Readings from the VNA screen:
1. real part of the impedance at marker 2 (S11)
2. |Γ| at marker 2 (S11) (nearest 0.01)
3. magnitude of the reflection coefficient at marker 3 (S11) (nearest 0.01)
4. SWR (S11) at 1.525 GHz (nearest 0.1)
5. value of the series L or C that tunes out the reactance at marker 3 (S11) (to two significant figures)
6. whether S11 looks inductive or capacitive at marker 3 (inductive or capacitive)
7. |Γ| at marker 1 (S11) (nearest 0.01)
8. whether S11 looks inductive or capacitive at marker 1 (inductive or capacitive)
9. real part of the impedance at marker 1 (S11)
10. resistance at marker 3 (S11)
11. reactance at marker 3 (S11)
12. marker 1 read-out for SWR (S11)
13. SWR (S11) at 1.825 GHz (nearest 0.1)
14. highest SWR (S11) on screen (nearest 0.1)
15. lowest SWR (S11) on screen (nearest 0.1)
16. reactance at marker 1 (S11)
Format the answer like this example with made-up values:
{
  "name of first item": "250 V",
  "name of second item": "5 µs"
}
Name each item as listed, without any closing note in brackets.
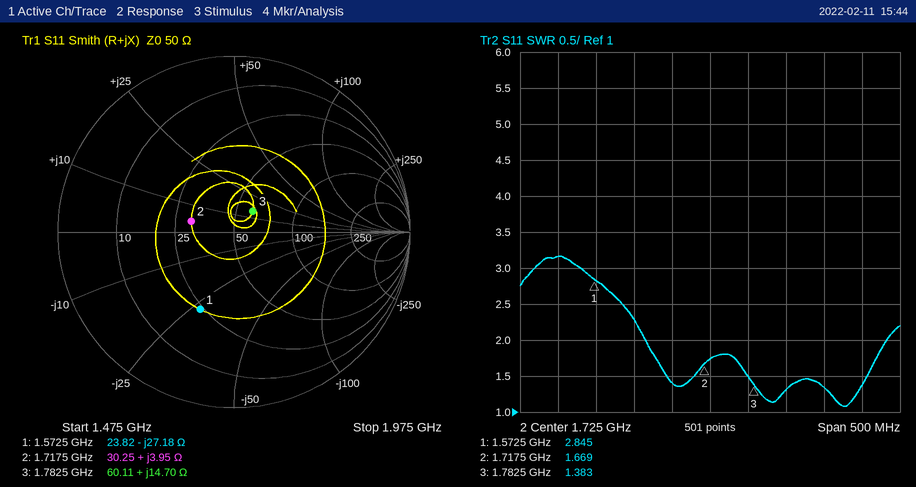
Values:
{
  "real part of the impedance at marker 2": "30.25 Ω",
  "|Γ| at marker 2 (S11)": "0.25",
  "magnitude of the reflection coefficient at marker 3 (S11)": "0.16",
  "SWR (S11) at 1.525 GHz": "3.2",
  "value of the series L or C that tunes out the reactance at marker 3 (S11)": "6.1 pF",
  "whether S11 looks inductive or capacitive at marker 3": "inductive",
  "|Γ| at marker 1 (S11)": "0.48",
  "whether S11 looks inductive or capacitive at marker 1": "capacitive",
  "real part of the impedance at marker 1": "23.82 Ω",
  "resistance at marker 3": "60.11 Ω",
  "reactance at marker 3": "+14.70 Ω",
  "marker 1 read-out for SWR": "2.845",
  "SWR (S11) at 1.825 GHz": "1.3",
  "highest SWR (S11) on screen": "3.2",
  "lowest SWR (S11) on screen": "1.1",
  "reactance at marker 1": "-27.18 Ω"
}
